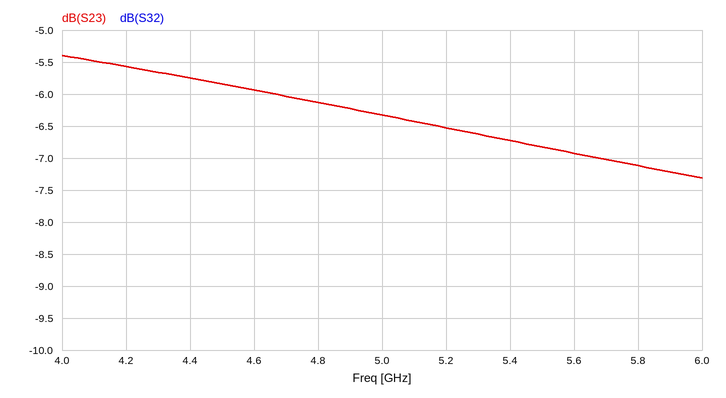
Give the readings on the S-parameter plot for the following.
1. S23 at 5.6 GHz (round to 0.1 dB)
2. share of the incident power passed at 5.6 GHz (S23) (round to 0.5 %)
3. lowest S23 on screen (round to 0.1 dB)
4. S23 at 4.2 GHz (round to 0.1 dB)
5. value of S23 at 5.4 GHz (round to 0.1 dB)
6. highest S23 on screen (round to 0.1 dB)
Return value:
-6.9 dB
20.5 %
-7.3 dB
-5.6 dB
-6.7 dB
-5.4 dB
